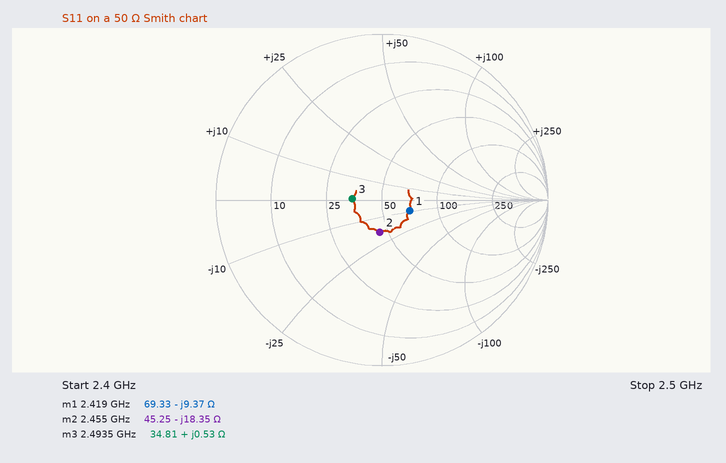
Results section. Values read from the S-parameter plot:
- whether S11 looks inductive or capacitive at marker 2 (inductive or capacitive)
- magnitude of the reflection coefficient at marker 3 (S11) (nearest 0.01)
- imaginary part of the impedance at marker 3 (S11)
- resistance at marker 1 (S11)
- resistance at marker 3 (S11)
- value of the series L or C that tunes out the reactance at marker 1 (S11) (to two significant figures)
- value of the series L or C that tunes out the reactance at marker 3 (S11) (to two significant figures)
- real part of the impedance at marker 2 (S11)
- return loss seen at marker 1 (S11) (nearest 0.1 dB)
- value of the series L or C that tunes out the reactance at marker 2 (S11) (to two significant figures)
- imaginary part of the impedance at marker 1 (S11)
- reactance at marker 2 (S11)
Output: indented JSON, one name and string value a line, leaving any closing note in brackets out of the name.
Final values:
{
  "whether S11 looks inductive or capacitive at marker 2": "capacitive",
  "magnitude of the reflection coefficient at marker 3 (S11)": "0.18",
  "imaginary part of the impedance at marker 3": "+0.53 Ω",
  "resistance at marker 1": "69.33 Ω",
  "resistance at marker 3": "34.81 Ω",
  "value of the series L or C that tunes out the reactance at marker 1 (S11)": "620 pH",
  "value of the series L or C that tunes out the reactance at marker 3 (S11)": "120 pF",
  "real part of the impedance at marker 2": "45.25 Ω",
  "return loss seen at marker 1 (S11)": "14.9 dB",
  "value of the series L or C that tunes out the reactance at marker 2 (S11)": "1.2 nH",
  "imaginary part of the impedance at marker 1": "-9.37 Ω",
  "reactance at marker 2": "-18.35 Ω"
}
